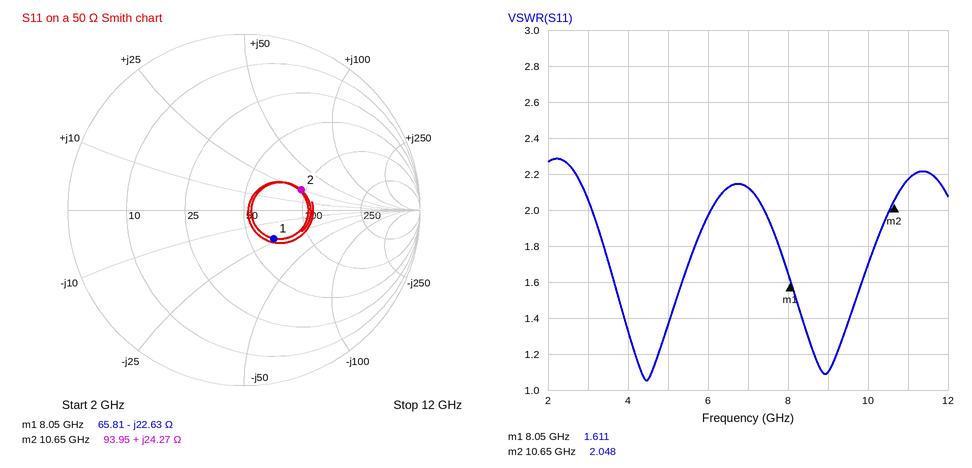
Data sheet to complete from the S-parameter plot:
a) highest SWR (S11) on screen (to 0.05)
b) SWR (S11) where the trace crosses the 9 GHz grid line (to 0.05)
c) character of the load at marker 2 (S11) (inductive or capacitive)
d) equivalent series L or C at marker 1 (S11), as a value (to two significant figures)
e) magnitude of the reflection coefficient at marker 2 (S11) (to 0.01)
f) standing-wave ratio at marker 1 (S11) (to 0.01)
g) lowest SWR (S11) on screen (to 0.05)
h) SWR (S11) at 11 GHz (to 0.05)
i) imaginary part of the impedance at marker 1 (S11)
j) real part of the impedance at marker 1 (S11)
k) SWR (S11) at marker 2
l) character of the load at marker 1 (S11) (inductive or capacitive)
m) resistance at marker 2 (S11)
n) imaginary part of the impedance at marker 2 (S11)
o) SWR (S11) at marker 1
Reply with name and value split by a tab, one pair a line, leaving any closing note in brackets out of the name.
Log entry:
highest SWR (S11) on screen	2.30
SWR (S11) where the trace crosses the 9 GHz grid line	1.10
character of the load at marker 2 (S11)	inductive
equivalent series L or C at marker 1 (S11), as a value	870 fF
magnitude of the reflection coefficient at marker 2 (S11)	0.34
standing-wave ratio at marker 1 (S11)	1.61
lowest SWR (S11) on screen	1.05
SWR (S11) at 11 GHz	2.15
imaginary part of the impedance at marker 1	-22.63 Ω
real part of the impedance at marker 1	65.81 Ω
SWR (S11) at marker 2	2.048
character of the load at marker 1 (S11)	capacitive
resistance at marker 2	93.95 Ω
imaginary part of the impedance at marker 2	+24.27 Ω
SWR (S11) at marker 1	1.611
